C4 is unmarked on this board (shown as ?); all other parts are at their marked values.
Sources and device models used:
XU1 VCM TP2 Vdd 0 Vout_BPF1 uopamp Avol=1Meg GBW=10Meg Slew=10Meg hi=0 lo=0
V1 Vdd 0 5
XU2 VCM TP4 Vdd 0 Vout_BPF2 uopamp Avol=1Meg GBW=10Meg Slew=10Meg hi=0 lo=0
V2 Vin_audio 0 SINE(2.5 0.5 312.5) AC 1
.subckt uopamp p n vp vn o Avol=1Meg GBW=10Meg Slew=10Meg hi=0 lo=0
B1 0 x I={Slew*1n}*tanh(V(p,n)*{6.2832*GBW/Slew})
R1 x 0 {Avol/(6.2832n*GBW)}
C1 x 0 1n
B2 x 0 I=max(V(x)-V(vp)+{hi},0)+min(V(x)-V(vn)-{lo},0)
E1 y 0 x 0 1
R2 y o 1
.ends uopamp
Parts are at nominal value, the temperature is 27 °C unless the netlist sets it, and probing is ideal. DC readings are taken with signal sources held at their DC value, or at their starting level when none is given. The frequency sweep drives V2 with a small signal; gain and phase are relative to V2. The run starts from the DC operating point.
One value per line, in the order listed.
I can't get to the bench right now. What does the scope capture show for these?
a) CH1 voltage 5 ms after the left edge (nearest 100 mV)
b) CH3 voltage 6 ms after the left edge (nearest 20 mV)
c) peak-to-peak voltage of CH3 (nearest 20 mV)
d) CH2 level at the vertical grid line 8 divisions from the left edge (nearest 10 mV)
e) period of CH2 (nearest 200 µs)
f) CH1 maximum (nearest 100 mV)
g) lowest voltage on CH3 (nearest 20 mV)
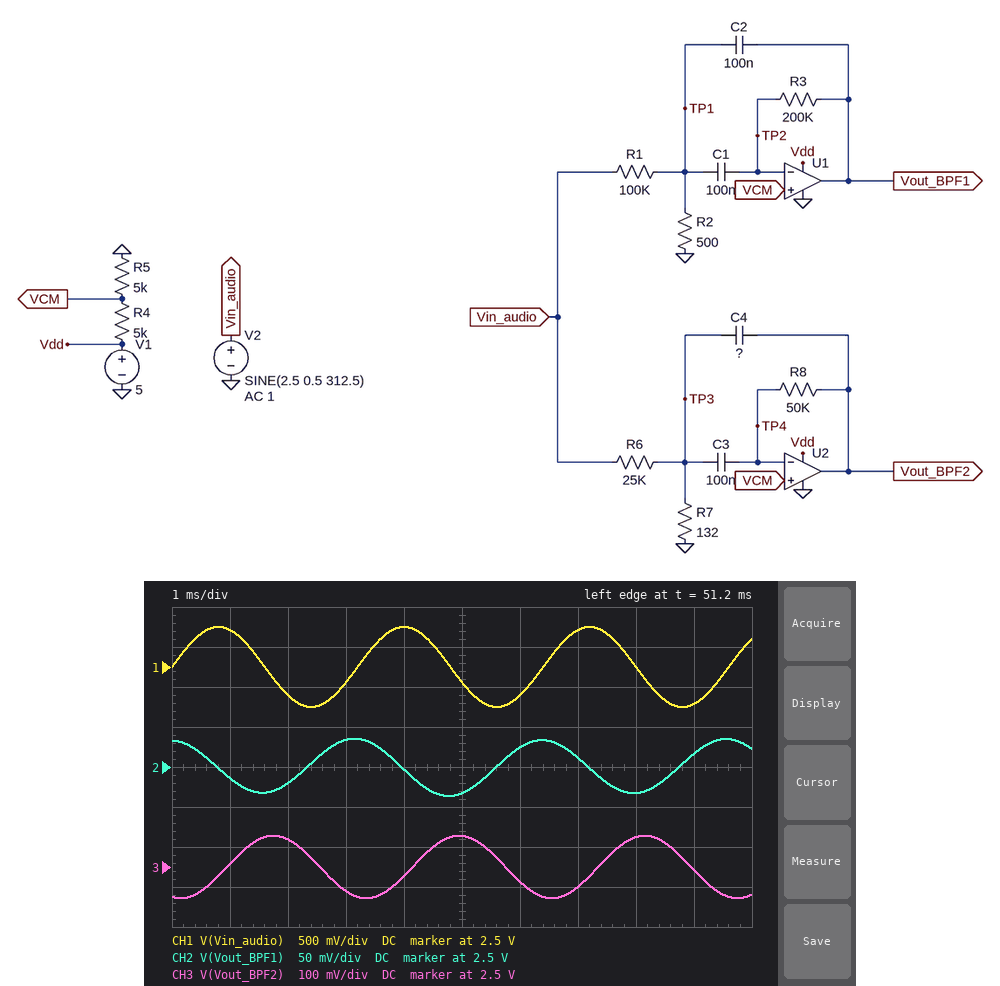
2.3 V
2.46 V
160 mV
2.47 V
3.2 ms
3.0 V
2.42 V
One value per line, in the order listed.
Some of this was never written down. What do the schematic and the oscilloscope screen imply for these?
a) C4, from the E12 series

270 nF
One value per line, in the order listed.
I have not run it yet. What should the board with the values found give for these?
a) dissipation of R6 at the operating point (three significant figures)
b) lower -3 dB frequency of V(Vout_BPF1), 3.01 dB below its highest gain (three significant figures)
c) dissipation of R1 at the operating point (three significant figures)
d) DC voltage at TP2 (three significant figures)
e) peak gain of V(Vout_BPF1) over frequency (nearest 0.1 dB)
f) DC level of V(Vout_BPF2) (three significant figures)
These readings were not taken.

247 µW
152 Hz
61.9 µW
2.50 V
0 dB
2.50 V
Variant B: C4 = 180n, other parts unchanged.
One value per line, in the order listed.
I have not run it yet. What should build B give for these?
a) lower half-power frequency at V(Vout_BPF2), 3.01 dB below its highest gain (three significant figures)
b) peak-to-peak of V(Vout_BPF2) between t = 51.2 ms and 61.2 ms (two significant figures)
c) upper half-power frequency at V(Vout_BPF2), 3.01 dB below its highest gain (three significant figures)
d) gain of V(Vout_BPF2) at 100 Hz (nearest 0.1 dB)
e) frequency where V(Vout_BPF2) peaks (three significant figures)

439 Hz
94 mV
488 Hz
-35.2 dB
463 Hz
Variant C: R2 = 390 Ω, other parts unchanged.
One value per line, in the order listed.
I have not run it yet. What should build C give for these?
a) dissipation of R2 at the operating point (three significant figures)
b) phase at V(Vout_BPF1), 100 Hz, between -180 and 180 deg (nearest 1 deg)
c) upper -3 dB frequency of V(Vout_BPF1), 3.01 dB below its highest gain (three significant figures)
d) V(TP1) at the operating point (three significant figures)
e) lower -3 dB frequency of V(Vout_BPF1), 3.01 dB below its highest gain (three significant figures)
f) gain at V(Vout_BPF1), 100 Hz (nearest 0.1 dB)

242 nW
-94 deg
189 Hz
9.71 mV
173 Hz
-23.1 dB
